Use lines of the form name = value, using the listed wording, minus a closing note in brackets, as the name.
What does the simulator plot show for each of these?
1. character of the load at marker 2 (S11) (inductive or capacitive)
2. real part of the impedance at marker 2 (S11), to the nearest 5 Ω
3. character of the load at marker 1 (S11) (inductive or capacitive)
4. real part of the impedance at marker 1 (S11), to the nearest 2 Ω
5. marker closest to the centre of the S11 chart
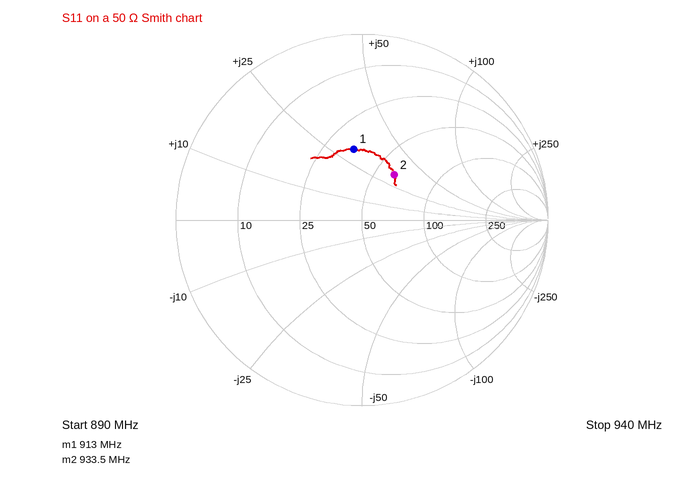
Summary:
character of the load at marker 2 (S11) = inductive
real part of the impedance at marker 2 (S11), to the nearest 5 Ω = 60 Ω
character of the load at marker 1 (S11) = inductive
real part of the impedance at marker 1 (S11), to the nearest 2 Ω = 34 Ω
marker closest to the centre of the S11 chart = marker 2
